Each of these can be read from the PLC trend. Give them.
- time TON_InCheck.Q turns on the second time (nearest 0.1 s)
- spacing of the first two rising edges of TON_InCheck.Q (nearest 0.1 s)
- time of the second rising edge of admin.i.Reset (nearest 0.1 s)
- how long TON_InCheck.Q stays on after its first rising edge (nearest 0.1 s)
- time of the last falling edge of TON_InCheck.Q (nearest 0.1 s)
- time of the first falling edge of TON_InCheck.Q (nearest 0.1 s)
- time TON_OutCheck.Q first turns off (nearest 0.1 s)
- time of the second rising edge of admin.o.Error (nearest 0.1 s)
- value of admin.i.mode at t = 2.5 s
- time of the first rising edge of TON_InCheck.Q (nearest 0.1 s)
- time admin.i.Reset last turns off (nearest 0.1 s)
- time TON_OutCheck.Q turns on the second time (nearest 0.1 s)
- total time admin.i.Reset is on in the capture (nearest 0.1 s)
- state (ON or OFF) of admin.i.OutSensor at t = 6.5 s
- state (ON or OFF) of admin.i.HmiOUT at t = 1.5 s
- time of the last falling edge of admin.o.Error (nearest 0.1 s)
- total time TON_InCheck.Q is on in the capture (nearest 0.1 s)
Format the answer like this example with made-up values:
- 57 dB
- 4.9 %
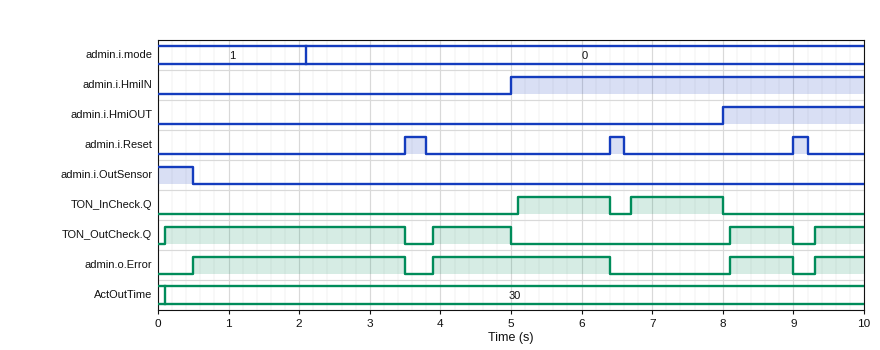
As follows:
- 6.7 s
- 1.6 s
- 6.4 s
- 1.3 s
- 8.0 s
- 6.4 s
- 3.5 s
- 3.9 s
- 0
- 5.1 s
- 9.2 s
- 3.9 s
- 0.7 s
- OFF
- OFF
- 9.0 s
- 2.6 s
